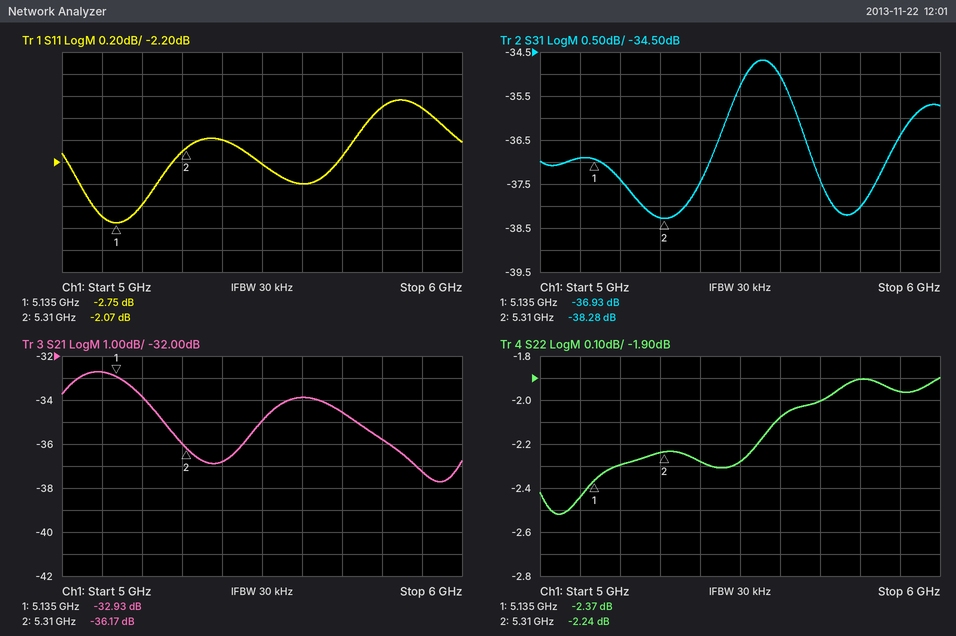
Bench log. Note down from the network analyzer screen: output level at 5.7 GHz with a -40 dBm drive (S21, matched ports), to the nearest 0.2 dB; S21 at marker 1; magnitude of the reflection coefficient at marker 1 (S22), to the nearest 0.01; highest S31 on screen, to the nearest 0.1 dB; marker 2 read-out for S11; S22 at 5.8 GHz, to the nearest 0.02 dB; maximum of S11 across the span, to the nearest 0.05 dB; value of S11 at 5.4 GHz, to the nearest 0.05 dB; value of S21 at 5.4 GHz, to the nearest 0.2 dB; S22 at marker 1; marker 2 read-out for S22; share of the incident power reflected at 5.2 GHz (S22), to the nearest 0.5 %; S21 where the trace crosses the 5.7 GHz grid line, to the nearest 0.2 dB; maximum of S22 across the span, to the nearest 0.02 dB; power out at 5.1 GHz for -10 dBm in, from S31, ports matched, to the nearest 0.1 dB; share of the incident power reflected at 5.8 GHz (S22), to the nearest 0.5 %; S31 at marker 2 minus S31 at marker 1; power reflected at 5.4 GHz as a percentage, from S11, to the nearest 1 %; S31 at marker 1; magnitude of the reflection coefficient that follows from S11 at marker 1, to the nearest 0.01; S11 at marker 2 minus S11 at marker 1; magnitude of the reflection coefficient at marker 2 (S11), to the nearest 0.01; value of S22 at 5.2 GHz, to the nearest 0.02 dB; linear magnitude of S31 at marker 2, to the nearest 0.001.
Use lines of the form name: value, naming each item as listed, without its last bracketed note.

output level at 5.7 GHz with a -40 dBm drive (S21, matched ports), to the nearest 0.2 dB: -74.6 dBm
S21 at marker 1: -32.93 dB
magnitude of the reflection coefficient at marker 1 (S22), to the nearest 0.01: 0.76
highest S31 on screen, to the nearest 0.1 dB: -34.7 dB
marker 2 read-out for S11: -2.07 dB
S22 at 5.8 GHz, to the nearest 0.02 dB: -1.90 dB
maximum of S11 across the span, to the nearest 0.05 dB: -1.65 dB
value of S11 at 5.4 GHz, to the nearest 0.05 dB: -2.00 dB
value of S21 at 5.4 GHz, to the nearest 0.2 dB: -36.8 dB
S22 at marker 1: -2.37 dB
marker 2 read-out for S22: -2.24 dB
share of the incident power reflected at 5.2 GHz (S22), to the nearest 0.5 %: 59.0 %
S21 where the trace crosses the 5.7 GHz grid line, to the nearest 0.2 dB: -34.6 dB
maximum of S22 across the span, to the nearest 0.02 dB: -1.90 dB
power out at 5.1 GHz for -10 dBm in, from S31, ports matched, to the nearest 0.1 dB: -46.9 dBm
share of the incident power reflected at 5.8 GHz (S22), to the nearest 0.5 %: 64.5 %
S31 at marker 2 minus S31 at marker 1: -1.35 dB
power reflected at 5.4 GHz as a percentage, from S11, to the nearest 1 %: 63 %
S31 at marker 1: -36.93 dB
magnitude of the reflection coefficient that follows from S11 at marker 1, to the nearest 0.01: 0.73
S11 at marker 2 minus S11 at marker 1: 0.68 dB
magnitude of the reflection coefficient at marker 2 (S11), to the nearest 0.01: 0.79
value of S22 at 5.2 GHz, to the nearest 0.02 dB: -2.30 dB
linear magnitude of S31 at marker 2, to the nearest 0.001: 0.012
